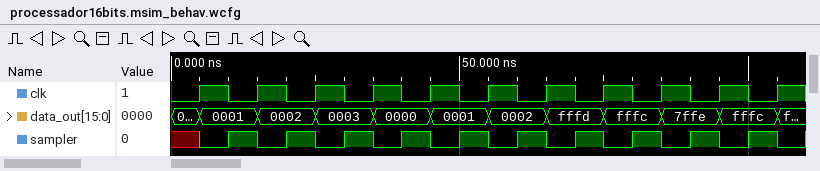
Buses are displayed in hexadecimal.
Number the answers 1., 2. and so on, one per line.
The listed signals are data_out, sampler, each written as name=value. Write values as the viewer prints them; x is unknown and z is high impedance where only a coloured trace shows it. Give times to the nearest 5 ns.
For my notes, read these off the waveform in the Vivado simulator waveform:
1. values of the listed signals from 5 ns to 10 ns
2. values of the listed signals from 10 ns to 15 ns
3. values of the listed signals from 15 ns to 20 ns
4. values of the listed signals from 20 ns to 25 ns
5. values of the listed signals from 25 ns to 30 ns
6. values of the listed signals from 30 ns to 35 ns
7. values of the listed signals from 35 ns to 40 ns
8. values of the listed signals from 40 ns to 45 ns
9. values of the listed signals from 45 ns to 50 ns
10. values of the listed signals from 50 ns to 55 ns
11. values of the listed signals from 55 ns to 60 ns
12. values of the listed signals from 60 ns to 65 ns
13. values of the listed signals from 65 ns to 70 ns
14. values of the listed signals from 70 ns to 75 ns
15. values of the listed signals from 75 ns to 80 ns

1. data_out=0001, sampler=0
2. data_out=0001, sampler=1
3. data_out=0002, sampler=0
4. data_out=0002, sampler=1
5. data_out=0003, sampler=0
6. data_out=0003, sampler=1
7. data_out=0000, sampler=0
8. data_out=0000, sampler=1
9. data_out=0001, sampler=0
10. data_out=0001, sampler=1
11. data_out=0002, sampler=0
12. data_out=0002, sampler=1
13. data_out=fffd, sampler=0
14. data_out=fffd, sampler=1
15. data_out=fffc, sampler=0
